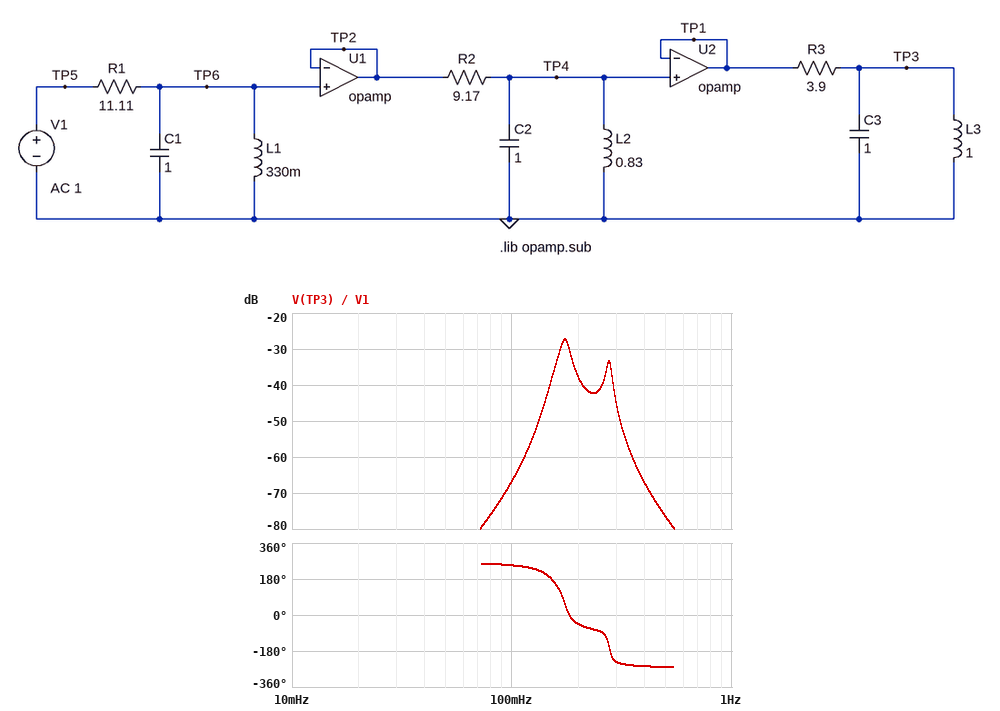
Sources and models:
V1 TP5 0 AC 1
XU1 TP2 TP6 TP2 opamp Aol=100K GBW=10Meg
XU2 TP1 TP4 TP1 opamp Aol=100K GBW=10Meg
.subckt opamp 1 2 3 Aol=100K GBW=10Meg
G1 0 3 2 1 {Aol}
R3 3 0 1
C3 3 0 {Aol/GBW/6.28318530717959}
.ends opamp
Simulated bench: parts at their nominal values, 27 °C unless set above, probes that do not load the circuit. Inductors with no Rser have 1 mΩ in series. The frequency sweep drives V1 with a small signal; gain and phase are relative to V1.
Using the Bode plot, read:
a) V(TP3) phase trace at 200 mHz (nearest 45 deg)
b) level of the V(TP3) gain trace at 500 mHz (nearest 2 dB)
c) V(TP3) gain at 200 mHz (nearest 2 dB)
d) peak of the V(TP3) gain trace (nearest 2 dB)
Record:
-45 deg
-76 dB
-38 dB
-28 dB
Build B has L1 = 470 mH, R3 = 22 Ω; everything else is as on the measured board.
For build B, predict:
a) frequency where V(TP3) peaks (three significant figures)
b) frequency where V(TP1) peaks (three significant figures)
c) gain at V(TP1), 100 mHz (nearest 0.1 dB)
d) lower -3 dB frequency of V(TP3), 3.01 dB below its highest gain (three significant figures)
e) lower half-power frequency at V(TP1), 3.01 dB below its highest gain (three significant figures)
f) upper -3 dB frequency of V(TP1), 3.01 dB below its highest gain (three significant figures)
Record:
160 mHz
231 mHz
-51.2 dB
157 mHz
223 mHz
238 mHz
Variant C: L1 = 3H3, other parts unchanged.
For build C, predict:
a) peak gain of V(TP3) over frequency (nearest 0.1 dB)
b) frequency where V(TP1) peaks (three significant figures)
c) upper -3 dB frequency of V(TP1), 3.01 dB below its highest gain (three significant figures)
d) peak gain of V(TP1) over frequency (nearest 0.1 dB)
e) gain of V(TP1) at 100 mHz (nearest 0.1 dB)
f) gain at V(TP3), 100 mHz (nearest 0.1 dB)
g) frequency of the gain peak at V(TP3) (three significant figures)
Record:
-20.9 dB
174 mHz
182 mHz
-19.3 dB
-27.1 dB
-38.9 dB
172 mHz
